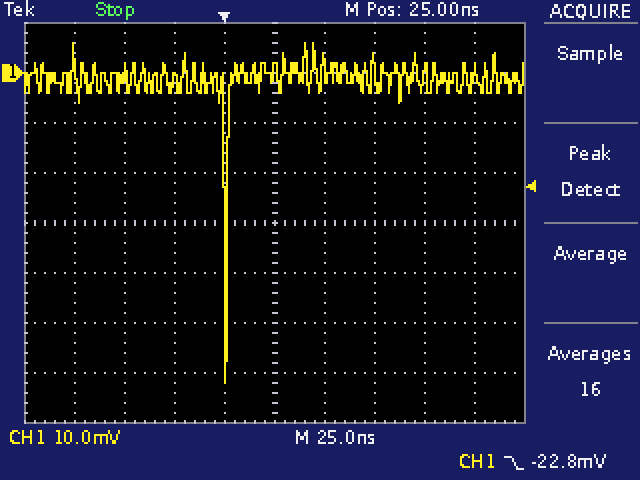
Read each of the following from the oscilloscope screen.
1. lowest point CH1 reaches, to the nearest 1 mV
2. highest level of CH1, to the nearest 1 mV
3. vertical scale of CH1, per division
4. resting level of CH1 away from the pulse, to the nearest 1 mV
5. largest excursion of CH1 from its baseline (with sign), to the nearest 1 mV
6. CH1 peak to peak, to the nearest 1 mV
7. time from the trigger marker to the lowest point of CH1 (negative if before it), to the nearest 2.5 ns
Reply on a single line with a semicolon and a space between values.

-62 mV; 6 mV; 10 mV; -1 mV; -61 mV; 68 mV; 0.0 ns
